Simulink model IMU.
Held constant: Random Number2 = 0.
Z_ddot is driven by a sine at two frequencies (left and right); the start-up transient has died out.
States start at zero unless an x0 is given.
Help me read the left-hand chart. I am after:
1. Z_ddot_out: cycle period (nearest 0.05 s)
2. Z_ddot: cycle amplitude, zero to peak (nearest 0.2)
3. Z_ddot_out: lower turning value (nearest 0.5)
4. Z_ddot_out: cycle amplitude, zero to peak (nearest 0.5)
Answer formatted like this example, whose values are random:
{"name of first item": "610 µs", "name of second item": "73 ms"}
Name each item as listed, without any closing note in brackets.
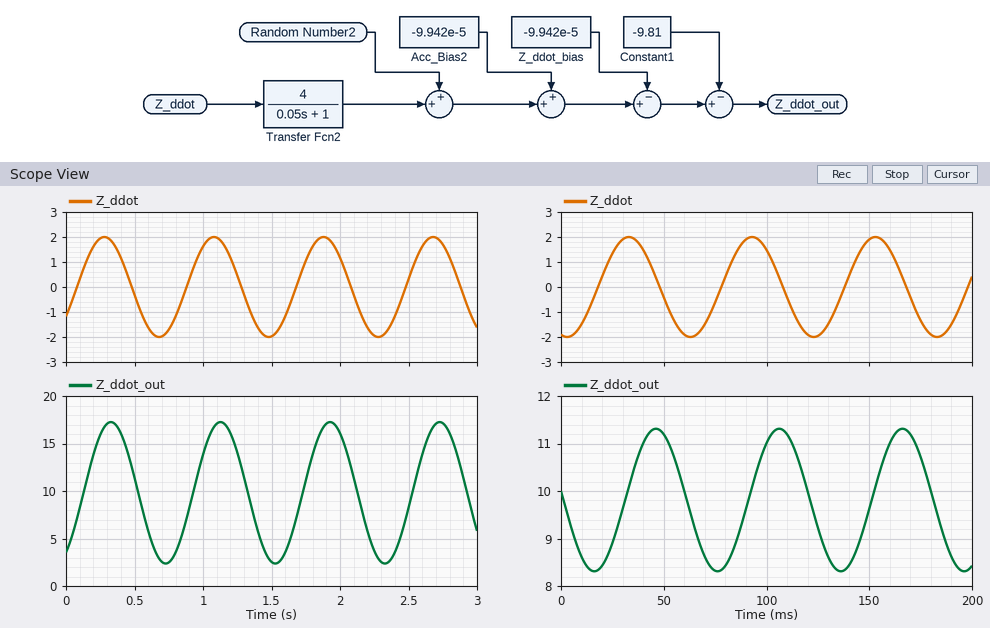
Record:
{"Z_ddot_out: cycle period": "0.80 s", "Z_ddot: cycle amplitude, zero to peak": "2.0", "Z_ddot_out: lower turning value": "2.5", "Z_ddot_out: cycle amplitude, zero to peak": "7.5"}
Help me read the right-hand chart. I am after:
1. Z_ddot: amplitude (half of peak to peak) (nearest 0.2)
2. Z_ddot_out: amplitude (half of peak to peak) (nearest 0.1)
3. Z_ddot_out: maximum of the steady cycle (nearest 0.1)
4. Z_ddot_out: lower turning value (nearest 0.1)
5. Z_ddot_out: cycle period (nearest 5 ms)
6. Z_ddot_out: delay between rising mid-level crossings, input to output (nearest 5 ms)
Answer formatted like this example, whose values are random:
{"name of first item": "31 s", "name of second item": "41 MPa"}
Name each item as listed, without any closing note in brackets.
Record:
{"Z_ddot: amplitude (half of peak to peak)": "2.0", "Z_ddot_out: amplitude (half of peak to peak)": "1.5", "Z_ddot_out: maximum of the steady cycle": "11.3", "Z_ddot_out: lower turning value": "8.3", "Z_ddot_out: cycle period": "60 ms", "Z_ddot_out: delay between rising mid-level crossings, input to output": "15 ms"}
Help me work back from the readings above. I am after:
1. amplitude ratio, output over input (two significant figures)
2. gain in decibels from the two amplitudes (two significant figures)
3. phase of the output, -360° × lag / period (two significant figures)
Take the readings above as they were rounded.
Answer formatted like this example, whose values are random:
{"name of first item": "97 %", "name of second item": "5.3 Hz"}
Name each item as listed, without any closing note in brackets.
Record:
{"amplitude ratio, output over input": "0.75", "gain in decibels from the two amplitudes": "-2.5 dB", "phase of the output, -360° × lag / period": "-90°"}
